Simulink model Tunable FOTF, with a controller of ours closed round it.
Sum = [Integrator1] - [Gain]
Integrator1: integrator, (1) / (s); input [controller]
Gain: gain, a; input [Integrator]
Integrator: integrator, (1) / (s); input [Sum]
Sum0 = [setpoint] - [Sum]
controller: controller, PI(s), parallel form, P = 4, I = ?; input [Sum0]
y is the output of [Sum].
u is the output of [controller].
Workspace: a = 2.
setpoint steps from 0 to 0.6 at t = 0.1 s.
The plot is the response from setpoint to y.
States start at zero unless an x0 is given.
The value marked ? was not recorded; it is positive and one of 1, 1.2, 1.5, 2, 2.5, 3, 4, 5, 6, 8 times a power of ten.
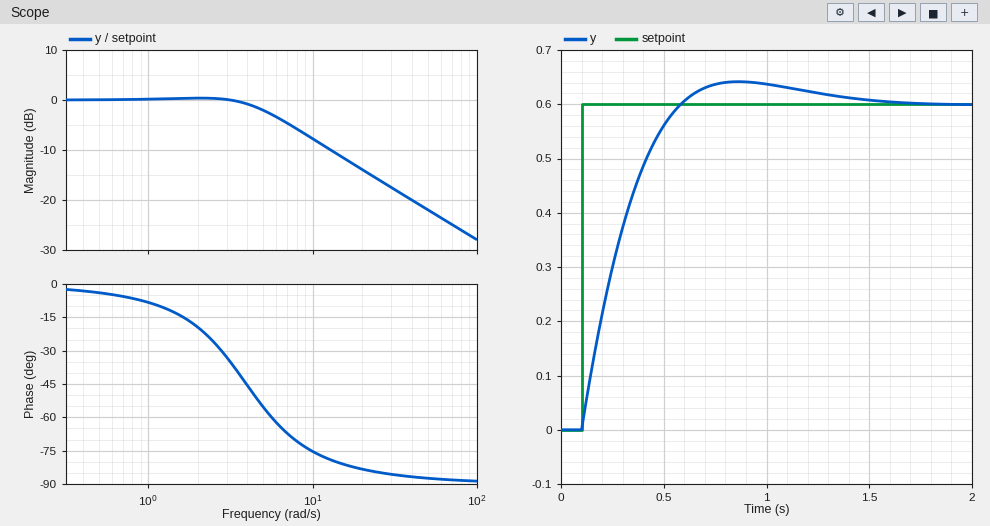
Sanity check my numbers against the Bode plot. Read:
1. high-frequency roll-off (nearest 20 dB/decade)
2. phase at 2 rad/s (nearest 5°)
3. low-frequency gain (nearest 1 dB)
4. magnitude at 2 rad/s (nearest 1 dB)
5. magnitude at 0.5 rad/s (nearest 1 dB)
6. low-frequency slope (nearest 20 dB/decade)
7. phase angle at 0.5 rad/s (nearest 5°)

-20 dB/decade
-20°
0 dB
0 dB
0 dB
0 dB/decade
-5°
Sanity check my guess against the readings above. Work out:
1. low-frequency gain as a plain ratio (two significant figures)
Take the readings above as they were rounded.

1.0
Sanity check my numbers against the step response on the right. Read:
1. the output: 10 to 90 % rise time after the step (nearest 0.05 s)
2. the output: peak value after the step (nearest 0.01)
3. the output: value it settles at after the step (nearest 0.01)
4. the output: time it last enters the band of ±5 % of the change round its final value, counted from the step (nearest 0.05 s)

0.35 s
0.64
0.60
1.00 s
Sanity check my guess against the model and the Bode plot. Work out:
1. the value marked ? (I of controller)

15
